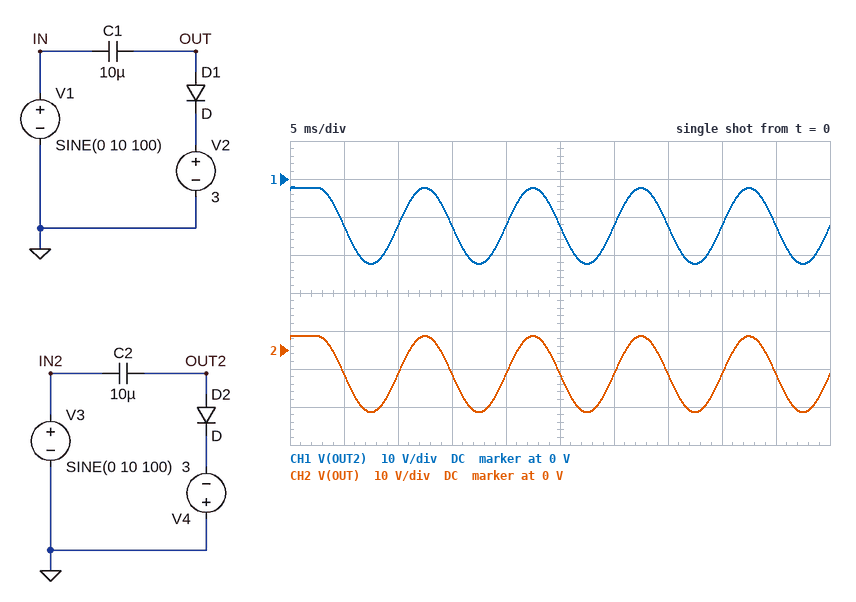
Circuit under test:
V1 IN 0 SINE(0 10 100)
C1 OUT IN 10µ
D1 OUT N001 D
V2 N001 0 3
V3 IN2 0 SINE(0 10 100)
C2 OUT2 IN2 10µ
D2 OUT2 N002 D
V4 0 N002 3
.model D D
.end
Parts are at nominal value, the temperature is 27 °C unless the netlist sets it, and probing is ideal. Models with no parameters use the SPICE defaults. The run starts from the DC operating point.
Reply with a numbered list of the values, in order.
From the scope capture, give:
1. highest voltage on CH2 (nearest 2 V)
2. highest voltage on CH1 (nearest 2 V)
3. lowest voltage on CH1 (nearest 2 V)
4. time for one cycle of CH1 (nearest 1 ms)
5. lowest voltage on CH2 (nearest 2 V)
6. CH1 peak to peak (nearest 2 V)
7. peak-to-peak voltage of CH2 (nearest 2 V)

1. 4 V
2. -2 V
3. -22 V
4. 10 ms
5. -16 V
6. 20 V
7. 20 V
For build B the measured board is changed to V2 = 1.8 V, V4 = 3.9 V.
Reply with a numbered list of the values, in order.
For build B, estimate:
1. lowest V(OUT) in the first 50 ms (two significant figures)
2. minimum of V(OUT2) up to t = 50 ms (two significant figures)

1. -18 V
2. -23 V
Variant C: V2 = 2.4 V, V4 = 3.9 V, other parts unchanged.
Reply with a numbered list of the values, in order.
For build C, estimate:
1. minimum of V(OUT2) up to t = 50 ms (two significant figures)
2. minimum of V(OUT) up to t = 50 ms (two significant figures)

1. -23 V
2. -17 V
